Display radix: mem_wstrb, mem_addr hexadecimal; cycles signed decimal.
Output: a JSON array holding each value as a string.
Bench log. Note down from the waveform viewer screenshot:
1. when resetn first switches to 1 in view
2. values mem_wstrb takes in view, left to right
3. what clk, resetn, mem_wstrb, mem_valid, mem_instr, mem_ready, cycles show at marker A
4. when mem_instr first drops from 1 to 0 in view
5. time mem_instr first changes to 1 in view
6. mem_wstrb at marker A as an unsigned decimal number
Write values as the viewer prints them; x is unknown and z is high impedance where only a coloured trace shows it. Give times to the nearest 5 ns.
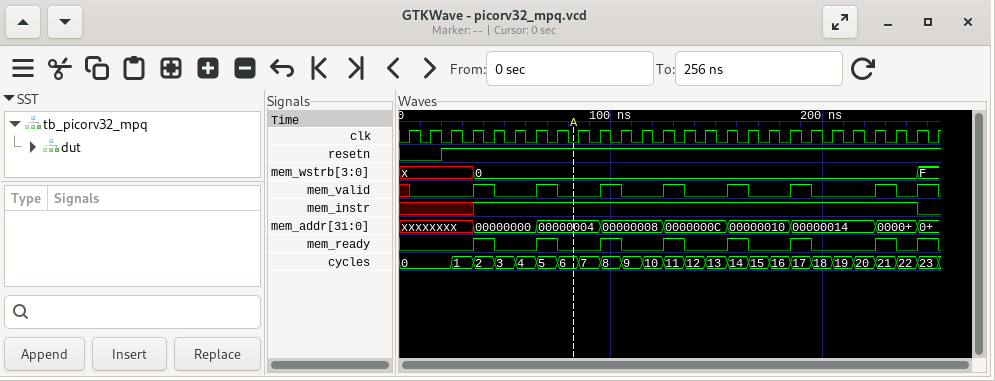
["20 ns", "x, 0, F", "clk=0, resetn=1, mem_wstrb=0, mem_valid=0, mem_instr=1, mem_ready=0, cycles=6", "245 ns", "35 ns", "0"]
